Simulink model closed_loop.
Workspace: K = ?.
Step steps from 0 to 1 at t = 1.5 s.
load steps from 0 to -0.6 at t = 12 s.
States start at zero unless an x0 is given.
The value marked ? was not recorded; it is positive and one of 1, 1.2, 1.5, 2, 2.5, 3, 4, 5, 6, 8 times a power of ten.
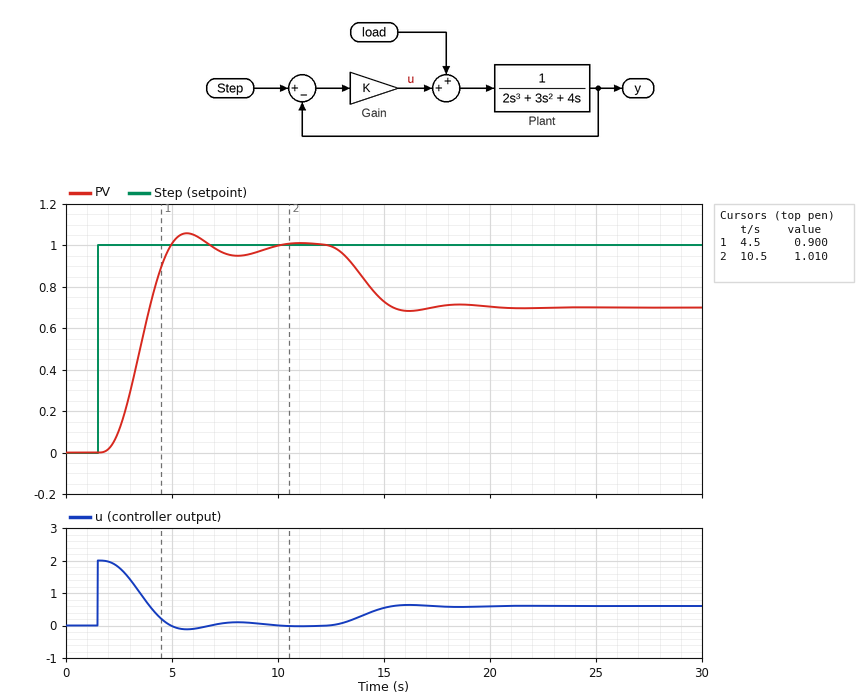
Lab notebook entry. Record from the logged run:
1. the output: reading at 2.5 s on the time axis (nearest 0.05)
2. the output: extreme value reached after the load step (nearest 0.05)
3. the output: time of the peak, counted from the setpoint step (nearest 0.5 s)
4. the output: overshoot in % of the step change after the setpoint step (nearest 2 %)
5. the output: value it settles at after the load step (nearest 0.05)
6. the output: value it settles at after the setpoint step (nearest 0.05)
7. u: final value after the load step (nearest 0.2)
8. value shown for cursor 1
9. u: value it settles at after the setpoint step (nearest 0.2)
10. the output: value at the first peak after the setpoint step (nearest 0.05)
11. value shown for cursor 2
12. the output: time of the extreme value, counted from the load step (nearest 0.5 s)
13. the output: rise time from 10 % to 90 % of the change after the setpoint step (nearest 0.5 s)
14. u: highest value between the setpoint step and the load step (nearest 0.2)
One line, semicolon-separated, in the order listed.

0.10; 0.70; 4.0 s; 6 %; 0.70; 1.00; 0.6; 0.900; 0.0; 1.05; 1.010; 4.0 s; 2.0 s; 2.0
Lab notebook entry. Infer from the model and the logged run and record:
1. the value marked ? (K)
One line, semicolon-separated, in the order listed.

2
